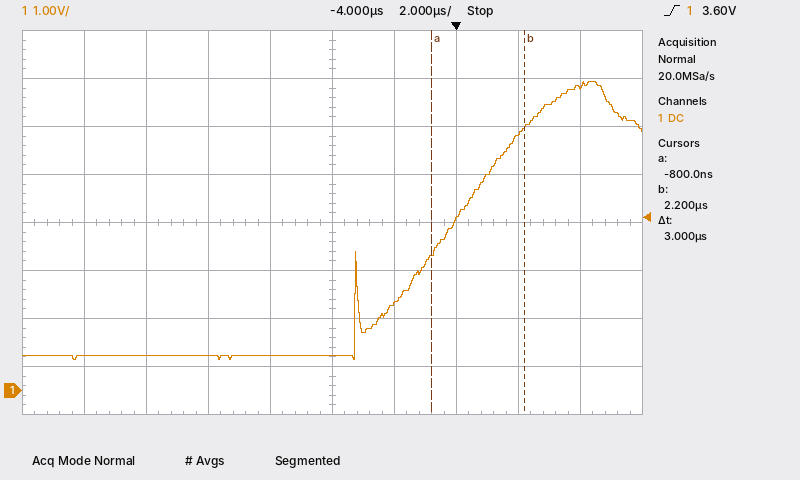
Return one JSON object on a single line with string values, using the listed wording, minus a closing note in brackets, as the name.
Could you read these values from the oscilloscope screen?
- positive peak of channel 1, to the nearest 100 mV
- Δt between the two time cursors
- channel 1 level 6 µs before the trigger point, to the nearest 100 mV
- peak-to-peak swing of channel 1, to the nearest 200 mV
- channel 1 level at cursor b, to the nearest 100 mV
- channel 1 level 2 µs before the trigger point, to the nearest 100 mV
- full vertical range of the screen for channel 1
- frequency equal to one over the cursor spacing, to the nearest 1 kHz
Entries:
{"positive peak of channel 1, to the nearest 100 mV": "6.4 V", "Δt between the two time cursors": "3 µs", "channel 1 level 6 µs before the trigger point, to the nearest 100 mV": "700 mV", "peak-to-peak swing of channel 1, to the nearest 200 mV": "5.8 V", "channel 1 level at cursor b, to the nearest 100 mV": "5.5 V", "channel 1 level 2 µs before the trigger point, to the nearest 100 mV": "1.8 V", "full vertical range of the screen for channel 1": "8 V", "frequency equal to one over the cursor spacing, to the nearest 1 kHz": "333 kHz"}
